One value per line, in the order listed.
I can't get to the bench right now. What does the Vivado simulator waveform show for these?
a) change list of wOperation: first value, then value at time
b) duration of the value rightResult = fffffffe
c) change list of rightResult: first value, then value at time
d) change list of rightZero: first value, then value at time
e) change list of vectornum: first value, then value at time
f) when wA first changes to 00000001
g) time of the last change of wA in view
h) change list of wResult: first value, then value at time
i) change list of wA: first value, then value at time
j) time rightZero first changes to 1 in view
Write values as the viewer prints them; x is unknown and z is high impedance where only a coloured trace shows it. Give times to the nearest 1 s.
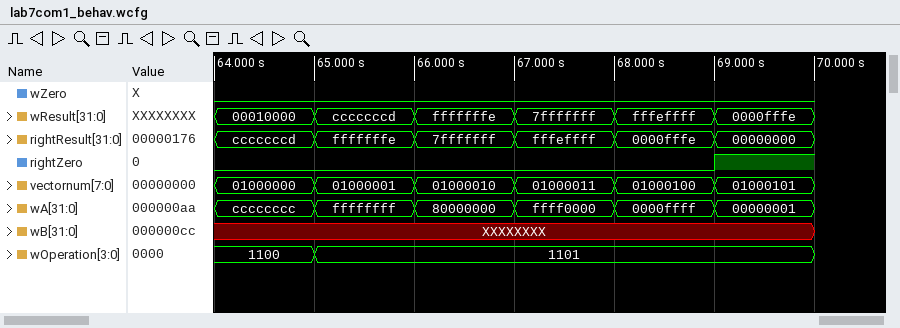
1100, 1101 at 65 s
1 s
cccccccd, fffffffe at 65 s, 7fffffff at 66 s, fffeffff at 67 s, 0000fffe at 68 s, 00000000 at 69 s
0, 1 at 69 s
01000000, 01000001 at 65 s, 01000010 at 66 s, 01000011 at 67 s, 01000100 at 68 s, 01000101 at 69 s
69 s
69 s
00010000, cccccccd at 65 s, fffffffe at 66 s, 7fffffff at 67 s, fffeffff at 68 s, 0000fffe at 69 s
cccccccc, ffffffff at 65 s, 80000000 at 66 s, ffff0000 at 67 s, 0000ffff at 68 s, 00000001 at 69 s
69 s
